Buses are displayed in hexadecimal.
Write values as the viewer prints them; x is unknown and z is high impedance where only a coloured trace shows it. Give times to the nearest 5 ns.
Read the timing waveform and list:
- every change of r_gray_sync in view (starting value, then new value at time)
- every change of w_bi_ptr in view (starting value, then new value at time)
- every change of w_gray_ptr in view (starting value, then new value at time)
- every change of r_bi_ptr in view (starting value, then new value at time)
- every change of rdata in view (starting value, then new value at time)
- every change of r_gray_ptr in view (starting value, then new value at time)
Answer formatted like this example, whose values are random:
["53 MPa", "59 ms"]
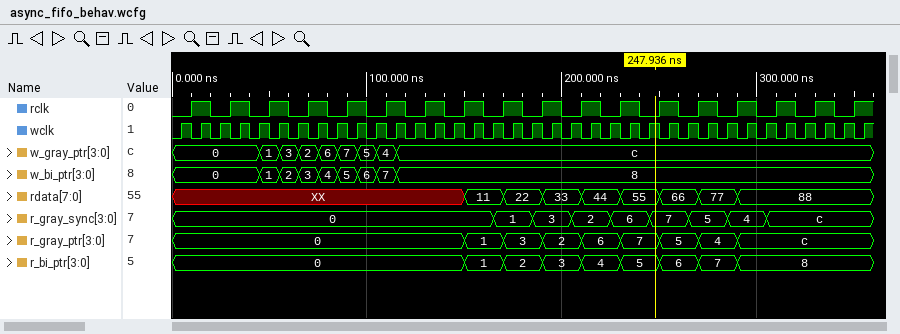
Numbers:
["0, 1 at 165 ns, 3 at 185 ns, 2 at 205 ns, 6 at 225 ns, 7 at 245 ns, 5 at 265 ns, 4 at 285 ns, c at 305 ns", "0, 1 at 45 ns, 2 at 55 ns, 3 at 65 ns, 4 at 75 ns, 5 at 85 ns, 6 at 95 ns, 7 at 105 ns, 8 at 115 ns", "0, 1 at 45 ns, 3 at 55 ns, 2 at 65 ns, 6 at 75 ns, 7 at 85 ns, 5 at 95 ns, 4 at 105 ns, c at 115 ns", "0, 1 at 150 ns, 2 at 170 ns, 3 at 190 ns, 4 at 210 ns, 5 at 230 ns, 6 at 250 ns, 7 at 270 ns, 8 at 290 ns", "XX, 11 at 150 ns, 22 at 170 ns, 33 at 190 ns, 44 at 210 ns, 55 at 230 ns, 66 at 250 ns, 77 at 270 ns, 88 at 290 ns", "0, 1 at 150 ns, 3 at 170 ns, 2 at 190 ns, 6 at 210 ns, 7 at 230 ns, 5 at 250 ns, 4 at 270 ns, c at 290 ns"]
